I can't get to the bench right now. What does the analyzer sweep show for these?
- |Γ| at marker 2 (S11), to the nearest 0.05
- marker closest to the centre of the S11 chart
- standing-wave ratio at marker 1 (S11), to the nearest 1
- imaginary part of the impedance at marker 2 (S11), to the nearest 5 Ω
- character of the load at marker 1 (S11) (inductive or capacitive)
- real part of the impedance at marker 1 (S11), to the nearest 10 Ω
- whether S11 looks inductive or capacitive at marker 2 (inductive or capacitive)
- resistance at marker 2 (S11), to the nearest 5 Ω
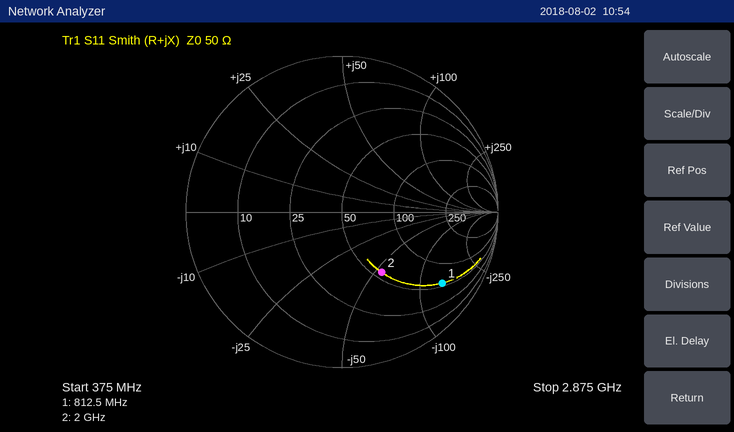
0.45
marker 2
8
-55 Ω
capacitive
60 Ω
capacitive
55 Ω
